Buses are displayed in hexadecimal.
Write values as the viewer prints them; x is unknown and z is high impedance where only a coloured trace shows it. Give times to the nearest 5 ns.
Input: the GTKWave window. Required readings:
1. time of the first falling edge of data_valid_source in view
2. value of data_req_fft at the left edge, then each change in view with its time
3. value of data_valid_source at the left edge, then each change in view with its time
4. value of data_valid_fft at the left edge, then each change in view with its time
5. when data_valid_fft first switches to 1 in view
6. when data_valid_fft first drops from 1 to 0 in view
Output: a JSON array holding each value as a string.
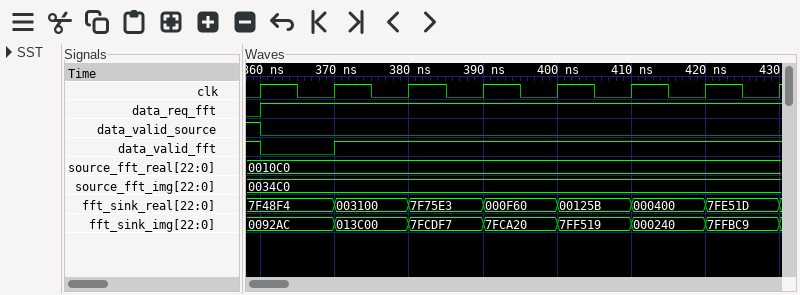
["360 ns", "0, 1 at 360 ns", "1, 0 at 360 ns", "1, 0 at 360 ns, 1 at 370 ns", "370 ns", "360 ns"]
